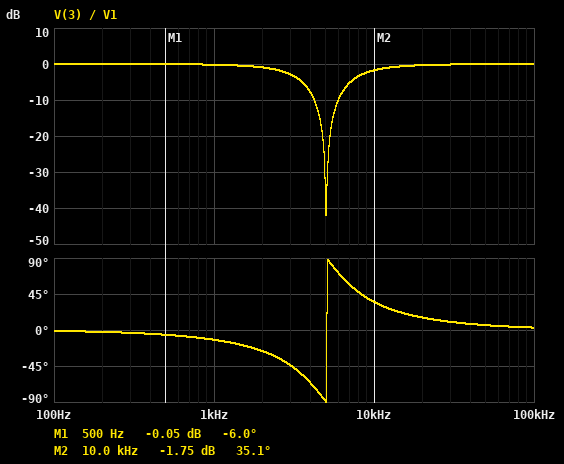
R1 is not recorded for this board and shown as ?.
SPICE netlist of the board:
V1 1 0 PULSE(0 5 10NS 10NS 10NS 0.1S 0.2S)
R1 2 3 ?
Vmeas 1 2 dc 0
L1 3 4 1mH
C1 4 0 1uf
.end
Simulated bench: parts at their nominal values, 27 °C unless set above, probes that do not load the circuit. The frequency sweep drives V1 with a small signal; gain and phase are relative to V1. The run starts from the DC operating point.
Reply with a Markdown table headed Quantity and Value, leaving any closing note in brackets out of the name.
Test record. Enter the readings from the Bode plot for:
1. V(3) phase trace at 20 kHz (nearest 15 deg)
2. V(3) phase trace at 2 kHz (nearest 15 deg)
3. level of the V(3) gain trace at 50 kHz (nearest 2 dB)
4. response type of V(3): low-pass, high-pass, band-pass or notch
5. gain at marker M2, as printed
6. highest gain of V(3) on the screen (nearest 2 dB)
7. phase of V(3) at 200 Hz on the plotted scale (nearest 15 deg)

| Quantity | Value |
|---|---|
| V(3) phase trace at 20 kHz | 15 deg |
| V(3) phase trace at 2 kHz | -30 deg |
| level of the V(3) gain trace at 50 kHz | 0 dB |
| response type of V(3): low-pass, high-pass, band-pass or notch | notch |
| gain at marker M2, as printed | -1.75 dB |
| highest gain of V(3) on the screen | 0 dB |
| phase of V(3) at 200 Hz on the plotted scale | 0 deg |
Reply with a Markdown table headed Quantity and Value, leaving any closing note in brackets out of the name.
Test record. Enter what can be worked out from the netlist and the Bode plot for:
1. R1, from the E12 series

| Quantity | Value |
|---|---|
| R1, from the E12 series | 33 Ω |
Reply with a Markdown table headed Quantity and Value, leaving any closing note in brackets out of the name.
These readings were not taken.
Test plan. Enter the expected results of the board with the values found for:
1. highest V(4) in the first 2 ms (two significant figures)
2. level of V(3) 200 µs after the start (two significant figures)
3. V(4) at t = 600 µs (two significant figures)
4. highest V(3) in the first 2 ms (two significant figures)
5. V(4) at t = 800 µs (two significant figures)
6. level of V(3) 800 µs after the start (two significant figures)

| Quantity | Value |
|---|---|
| highest V(4) in the first 2 ms | 5.7 V |
| level of V(3) 200 µs after the start | 5.2 V |
| V(4) at t = 600 µs | 5.0 V |
| highest V(3) in the first 2 ms | 5.4 V |
| V(4) at t = 800 µs | 5.0 V |
| level of V(3) 800 µs after the start | 5.0 V |
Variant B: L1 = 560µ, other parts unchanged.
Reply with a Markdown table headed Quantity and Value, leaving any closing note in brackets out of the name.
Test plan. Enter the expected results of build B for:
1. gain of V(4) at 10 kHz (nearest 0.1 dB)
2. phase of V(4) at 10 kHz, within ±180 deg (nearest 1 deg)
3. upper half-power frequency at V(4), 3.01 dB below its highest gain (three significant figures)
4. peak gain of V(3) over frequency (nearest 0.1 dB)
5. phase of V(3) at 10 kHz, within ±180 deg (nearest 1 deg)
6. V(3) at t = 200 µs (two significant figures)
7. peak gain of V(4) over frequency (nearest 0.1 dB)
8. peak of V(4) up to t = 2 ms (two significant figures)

| Quantity | Value |
|---|---|
| gain of V(4) at 10 kHz | -7.6 dB |
| phase of V(4) at 10 kHz, within ±180 deg | -120 deg |
| upper half-power frequency at V(4), 3.01 dB below its highest gain | 6.82 kHz |
| peak gain of V(3) over frequency | 0 dB |
| phase of V(3) at 10 kHz, within ±180 deg | 60 deg |
| V(3) at t = 200 µs | 5.0 V |
| peak gain of V(4) over frequency | 0 dB |
| peak of V(4) up to t = 2 ms | 5.2 V |
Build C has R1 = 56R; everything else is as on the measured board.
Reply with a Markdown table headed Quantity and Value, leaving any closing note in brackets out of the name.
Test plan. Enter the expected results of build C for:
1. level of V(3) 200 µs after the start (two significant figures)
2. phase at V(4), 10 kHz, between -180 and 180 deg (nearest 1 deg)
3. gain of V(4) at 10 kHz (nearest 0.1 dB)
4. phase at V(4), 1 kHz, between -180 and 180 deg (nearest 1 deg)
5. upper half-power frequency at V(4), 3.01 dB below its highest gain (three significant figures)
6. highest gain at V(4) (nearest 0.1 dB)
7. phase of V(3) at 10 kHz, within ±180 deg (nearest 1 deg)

| Quantity | Value |
|---|---|
| level of V(3) 200 µs after the start | 5.0 V |
| phase at V(4), 10 kHz, between -180 and 180 deg | -130 deg |
| gain of V(4) at 10 kHz | -13.2 dB |
| phase at V(4), 1 kHz, between -180 and 180 deg | -20 deg |
| upper half-power frequency at V(4), 3.01 dB below its highest gain | 3.84 kHz |
| highest gain at V(4) | 0 dB |
| phase of V(3) at 10 kHz, within ±180 deg | 50 deg |
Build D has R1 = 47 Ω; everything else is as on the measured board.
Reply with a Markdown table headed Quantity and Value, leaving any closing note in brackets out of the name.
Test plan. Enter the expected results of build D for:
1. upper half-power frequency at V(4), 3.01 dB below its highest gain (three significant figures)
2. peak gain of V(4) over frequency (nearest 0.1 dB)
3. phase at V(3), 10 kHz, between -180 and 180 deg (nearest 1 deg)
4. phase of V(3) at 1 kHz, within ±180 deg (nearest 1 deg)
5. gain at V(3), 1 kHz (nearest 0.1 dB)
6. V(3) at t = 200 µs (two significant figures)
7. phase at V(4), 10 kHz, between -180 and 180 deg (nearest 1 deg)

| Quantity | Value |
|---|---|
| upper half-power frequency at V(4), 3.01 dB below its highest gain | 4.78 kHz |
| peak gain of V(4) over frequency | 0 dB |
| phase at V(3), 10 kHz, between -180 and 180 deg | 45 deg |
| phase of V(3) at 1 kHz, within ±180 deg | -17 deg |
| gain at V(3), 1 kHz | -0.4 dB |
| V(3) at t = 200 µs | 5.1 V |
| phase at V(4), 10 kHz, between -180 and 180 deg | -135 deg |
